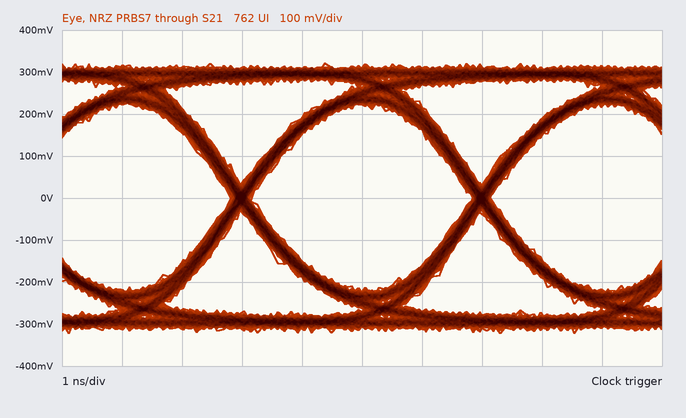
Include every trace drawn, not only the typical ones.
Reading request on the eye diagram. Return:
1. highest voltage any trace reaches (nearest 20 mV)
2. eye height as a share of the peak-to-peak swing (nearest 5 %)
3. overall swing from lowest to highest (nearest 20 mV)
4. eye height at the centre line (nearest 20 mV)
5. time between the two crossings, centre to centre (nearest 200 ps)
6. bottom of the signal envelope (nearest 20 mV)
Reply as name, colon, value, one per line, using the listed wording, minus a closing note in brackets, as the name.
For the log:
highest voltage any trace reaches: 320 mV
eye height as a share of the peak-to-peak swing: 70 %
overall swing from lowest to highest: 640 mV
eye height at the centre line: 440 mV
time between the two crossings, centre to centre: 4.0 ns
bottom of the signal envelope: -320 mV
